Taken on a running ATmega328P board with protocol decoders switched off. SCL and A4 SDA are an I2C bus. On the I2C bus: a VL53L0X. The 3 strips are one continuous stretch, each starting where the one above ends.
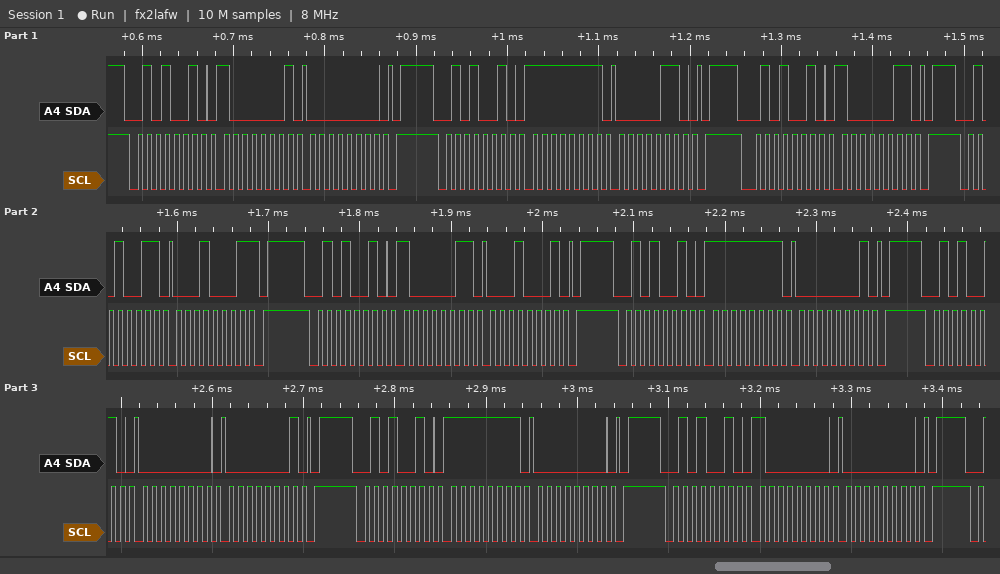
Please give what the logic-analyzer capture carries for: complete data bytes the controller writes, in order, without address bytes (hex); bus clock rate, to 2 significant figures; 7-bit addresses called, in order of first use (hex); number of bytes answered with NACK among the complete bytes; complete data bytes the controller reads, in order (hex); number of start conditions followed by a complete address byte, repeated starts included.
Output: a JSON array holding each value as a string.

["81 00 FF 06 83 83 11 FF 01 00 01 FF 00 80 00", "100 kHz", "0x29", "1", "11", "9"]
